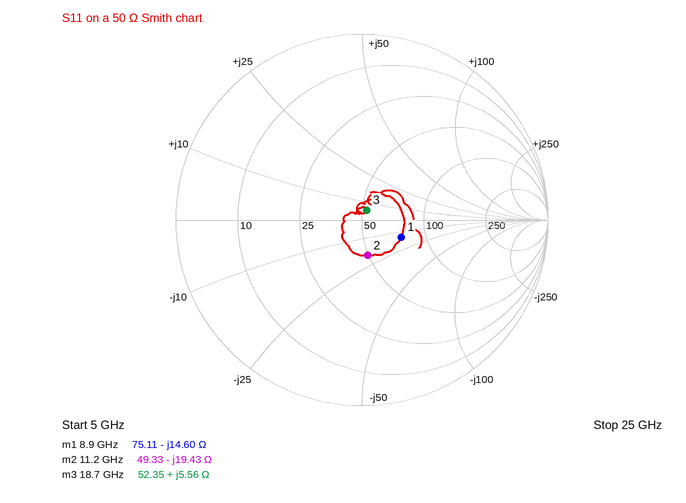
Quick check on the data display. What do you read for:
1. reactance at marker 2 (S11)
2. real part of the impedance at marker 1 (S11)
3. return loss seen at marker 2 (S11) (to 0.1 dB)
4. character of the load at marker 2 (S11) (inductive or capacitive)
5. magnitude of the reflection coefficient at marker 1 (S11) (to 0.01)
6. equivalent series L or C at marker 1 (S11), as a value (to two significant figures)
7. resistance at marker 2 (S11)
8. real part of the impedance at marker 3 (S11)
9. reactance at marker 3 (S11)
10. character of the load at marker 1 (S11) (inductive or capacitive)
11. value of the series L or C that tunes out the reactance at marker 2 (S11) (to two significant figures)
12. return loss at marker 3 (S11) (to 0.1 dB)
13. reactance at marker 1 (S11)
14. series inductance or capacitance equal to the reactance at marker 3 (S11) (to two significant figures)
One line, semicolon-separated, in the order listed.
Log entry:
-19.43 Ω; 75.11 Ω; 14.3 dB; capacitive; 0.23; 1.2 pF; 49.33 Ω; 52.35 Ω; +5.56 Ω; capacitive; 280 pH; 24.6 dB; -14.60 Ω; 47 pH
